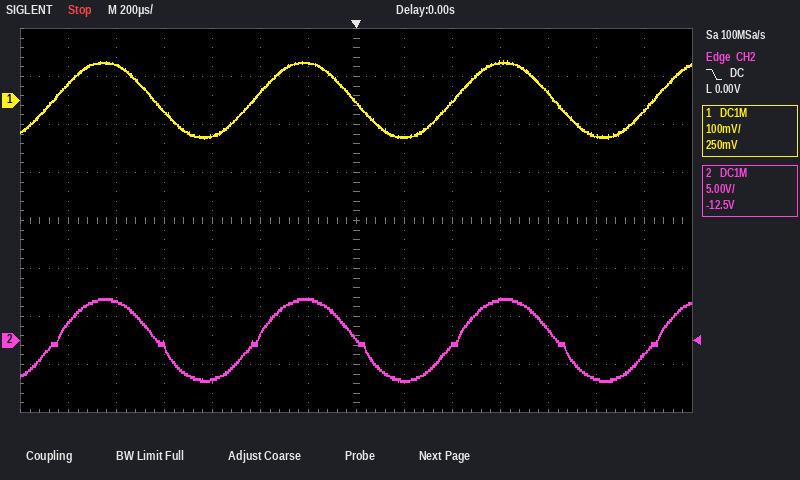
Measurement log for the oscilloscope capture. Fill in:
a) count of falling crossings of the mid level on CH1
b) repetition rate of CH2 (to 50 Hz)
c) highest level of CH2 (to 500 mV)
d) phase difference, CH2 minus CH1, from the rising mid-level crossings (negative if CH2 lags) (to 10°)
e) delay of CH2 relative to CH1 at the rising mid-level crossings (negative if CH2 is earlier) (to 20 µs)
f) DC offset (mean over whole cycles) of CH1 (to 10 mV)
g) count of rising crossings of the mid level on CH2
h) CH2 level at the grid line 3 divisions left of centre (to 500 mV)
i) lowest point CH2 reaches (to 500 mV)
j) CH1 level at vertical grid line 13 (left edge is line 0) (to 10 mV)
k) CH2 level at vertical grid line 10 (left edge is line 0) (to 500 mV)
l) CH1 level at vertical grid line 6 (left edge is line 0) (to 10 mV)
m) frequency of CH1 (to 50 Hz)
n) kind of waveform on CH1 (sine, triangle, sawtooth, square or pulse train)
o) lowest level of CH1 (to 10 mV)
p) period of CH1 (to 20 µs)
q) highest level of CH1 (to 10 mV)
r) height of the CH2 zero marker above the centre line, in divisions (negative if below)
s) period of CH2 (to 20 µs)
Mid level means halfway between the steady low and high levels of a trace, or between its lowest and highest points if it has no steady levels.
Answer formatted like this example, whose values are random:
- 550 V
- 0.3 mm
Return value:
- 3
- 1.20 kHz
- 4.5 V
- -10°
- +20 µs
- 0 mV
- 4
- -4.0 V
- -4.5 V
- -20 mV
- 4.0 V
- 80 mV
- 1.20 kHz
- sine
- -80 mV
- 840 µs
- 80 mV
- -2.5 div
- 840 µs
